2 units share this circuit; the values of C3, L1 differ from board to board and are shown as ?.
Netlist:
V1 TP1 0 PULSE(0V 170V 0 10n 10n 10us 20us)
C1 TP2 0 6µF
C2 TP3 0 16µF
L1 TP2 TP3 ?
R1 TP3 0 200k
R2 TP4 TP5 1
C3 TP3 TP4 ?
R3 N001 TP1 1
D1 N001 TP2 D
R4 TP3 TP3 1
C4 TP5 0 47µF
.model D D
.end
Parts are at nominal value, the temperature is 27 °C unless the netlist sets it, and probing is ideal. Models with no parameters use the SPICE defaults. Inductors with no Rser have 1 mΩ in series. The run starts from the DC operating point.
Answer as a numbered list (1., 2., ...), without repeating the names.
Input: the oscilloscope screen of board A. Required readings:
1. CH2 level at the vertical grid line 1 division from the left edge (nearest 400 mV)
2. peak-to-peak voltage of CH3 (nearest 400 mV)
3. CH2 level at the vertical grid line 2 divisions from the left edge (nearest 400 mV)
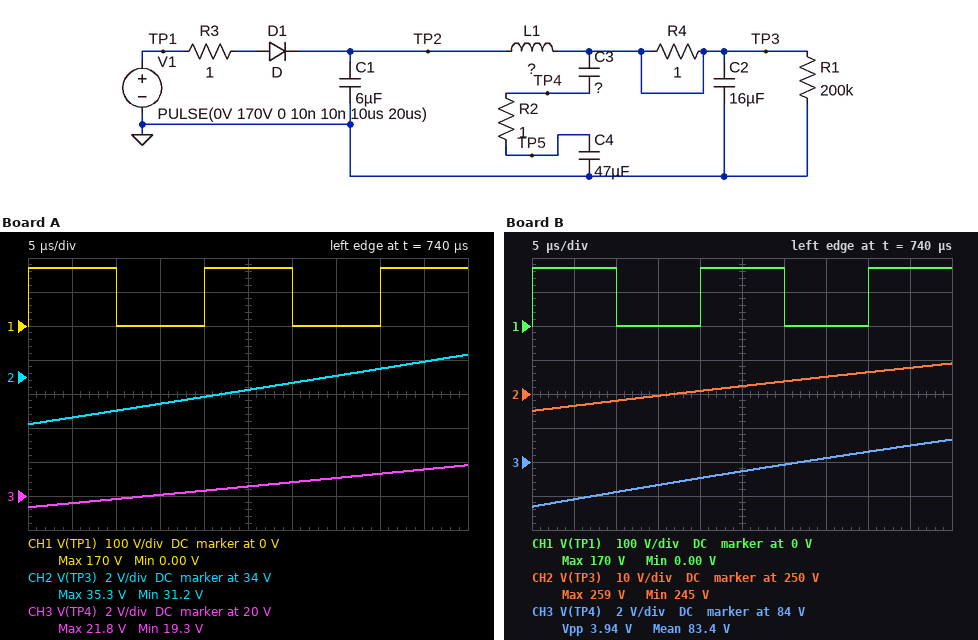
1. 31.6 V
2. 2.4 V
3. 32.0 V
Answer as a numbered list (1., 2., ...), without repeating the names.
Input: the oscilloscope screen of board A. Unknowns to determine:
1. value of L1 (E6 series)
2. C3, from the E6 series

1. 33 mH
2. 68 µF
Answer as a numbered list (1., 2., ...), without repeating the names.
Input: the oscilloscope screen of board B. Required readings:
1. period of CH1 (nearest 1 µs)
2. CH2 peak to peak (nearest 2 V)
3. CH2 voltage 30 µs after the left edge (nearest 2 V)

1. 20 µs
2. 14 V
3. 254 V
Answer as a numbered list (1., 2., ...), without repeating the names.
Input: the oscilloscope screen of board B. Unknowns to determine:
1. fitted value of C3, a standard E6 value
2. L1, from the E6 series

1. 22 µF
2. 3.3 mH
